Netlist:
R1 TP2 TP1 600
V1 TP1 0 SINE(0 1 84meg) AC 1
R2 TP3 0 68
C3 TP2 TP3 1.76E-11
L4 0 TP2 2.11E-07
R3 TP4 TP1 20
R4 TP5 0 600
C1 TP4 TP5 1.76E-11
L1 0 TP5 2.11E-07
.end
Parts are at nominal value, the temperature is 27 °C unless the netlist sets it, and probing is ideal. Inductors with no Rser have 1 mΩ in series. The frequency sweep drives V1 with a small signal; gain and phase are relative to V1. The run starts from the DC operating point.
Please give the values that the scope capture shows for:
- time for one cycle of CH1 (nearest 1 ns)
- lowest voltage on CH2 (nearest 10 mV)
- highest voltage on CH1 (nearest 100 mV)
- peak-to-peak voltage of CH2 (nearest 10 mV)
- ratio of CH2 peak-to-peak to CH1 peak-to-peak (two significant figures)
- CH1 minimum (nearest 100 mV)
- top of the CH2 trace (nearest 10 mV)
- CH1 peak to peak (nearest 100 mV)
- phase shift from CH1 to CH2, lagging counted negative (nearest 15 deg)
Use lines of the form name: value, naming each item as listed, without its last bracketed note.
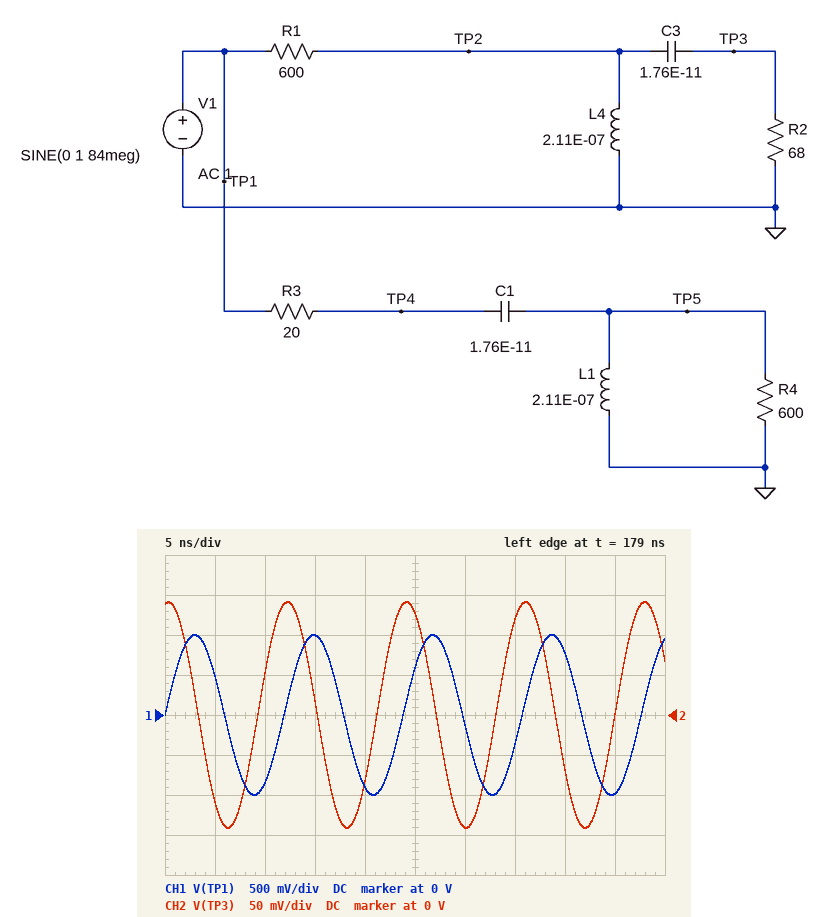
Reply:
time for one cycle of CH1: 12 ns
lowest voltage on CH2: -140 mV
highest voltage on CH1: 1.0 V
peak-to-peak voltage of CH2: 280 mV
ratio of CH2 peak-to-peak to CH1 peak-to-peak: 0.14
CH1 minimum: -1.0 V
top of the CH2 trace: 140 mV
CH1 peak to peak: 2.0 V
phase shift from CH1 to CH2, lagging counted negative: 75 deg
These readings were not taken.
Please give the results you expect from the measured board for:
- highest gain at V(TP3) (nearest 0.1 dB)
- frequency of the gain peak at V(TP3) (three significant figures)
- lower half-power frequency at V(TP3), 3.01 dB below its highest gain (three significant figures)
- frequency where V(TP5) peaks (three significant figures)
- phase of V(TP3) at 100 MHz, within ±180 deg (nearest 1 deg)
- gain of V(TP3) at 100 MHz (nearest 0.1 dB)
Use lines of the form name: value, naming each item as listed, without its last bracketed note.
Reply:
highest gain at V(TP3): -16.8 dB
frequency of the gain peak at V(TP3): 92.9 MHz
lower half-power frequency at V(TP3), 3.01 dB below its highest gain: 65.8 MHz
frequency where V(TP5) peaks: 84.0 MHz
phase of V(TP3) at 100 MHz, within ±180 deg: 57 deg
gain of V(TP3) at 100 MHz: -16.9 dB
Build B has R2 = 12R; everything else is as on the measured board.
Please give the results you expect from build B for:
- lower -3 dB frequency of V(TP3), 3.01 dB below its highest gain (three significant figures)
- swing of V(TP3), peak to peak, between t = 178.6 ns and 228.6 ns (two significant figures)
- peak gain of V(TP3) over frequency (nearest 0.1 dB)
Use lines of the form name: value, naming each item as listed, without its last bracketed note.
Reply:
lower -3 dB frequency of V(TP3), 3.01 dB below its highest gain: 73.3 MHz
swing of V(TP3), peak to peak, between t = 178.6 ns and 228.6 ns: 140 mV
peak gain of V(TP3) over frequency: -23.3 dB
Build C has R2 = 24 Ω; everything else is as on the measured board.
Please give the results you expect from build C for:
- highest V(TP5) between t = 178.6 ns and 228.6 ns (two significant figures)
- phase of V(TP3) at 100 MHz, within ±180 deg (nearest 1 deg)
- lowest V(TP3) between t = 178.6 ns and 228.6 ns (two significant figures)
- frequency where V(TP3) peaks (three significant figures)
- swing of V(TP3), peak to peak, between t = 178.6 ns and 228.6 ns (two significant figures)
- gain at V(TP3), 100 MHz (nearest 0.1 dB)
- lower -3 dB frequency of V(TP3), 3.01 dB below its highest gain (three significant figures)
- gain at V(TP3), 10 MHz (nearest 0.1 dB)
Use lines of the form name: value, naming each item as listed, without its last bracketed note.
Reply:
highest V(TP5) between t = 178.6 ns and 228.6 ns: 2.7 V
phase of V(TP3) at 100 MHz, within ±180 deg: 43 deg
lowest V(TP3) between t = 178.6 ns and 228.6 ns: -100 mV
frequency where V(TP3) peaks: 84.3 MHz
swing of V(TP3), peak to peak, between t = 178.6 ns and 228.6 ns: 200 mV
gain at V(TP3), 100 MHz: -21.7 dB
lower -3 dB frequency of V(TP3), 3.01 dB below its highest gain: 70.8 MHz
gain at V(TP3), 10 MHz: -64.5 dB
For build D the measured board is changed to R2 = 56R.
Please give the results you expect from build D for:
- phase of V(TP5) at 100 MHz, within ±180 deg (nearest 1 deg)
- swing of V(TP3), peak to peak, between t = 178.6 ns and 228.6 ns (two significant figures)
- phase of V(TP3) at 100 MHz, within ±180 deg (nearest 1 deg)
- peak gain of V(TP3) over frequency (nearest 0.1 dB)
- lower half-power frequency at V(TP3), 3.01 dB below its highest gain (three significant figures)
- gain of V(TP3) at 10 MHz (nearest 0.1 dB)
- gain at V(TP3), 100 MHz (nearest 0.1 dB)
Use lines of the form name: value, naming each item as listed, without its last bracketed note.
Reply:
phase of V(TP5) at 100 MHz, within ±180 deg: 41 deg
swing of V(TP3), peak to peak, between t = 178.6 ns and 228.6 ns: 270 mV
phase of V(TP3) at 100 MHz, within ±180 deg: 54 deg
peak gain of V(TP3) over frequency: -17.3 dB
lower half-power frequency at V(TP3), 3.01 dB below its highest gain: 66.6 MHz
gain of V(TP3) at 10 MHz: -57.2 dB
gain at V(TP3), 100 MHz: -17.6 dB
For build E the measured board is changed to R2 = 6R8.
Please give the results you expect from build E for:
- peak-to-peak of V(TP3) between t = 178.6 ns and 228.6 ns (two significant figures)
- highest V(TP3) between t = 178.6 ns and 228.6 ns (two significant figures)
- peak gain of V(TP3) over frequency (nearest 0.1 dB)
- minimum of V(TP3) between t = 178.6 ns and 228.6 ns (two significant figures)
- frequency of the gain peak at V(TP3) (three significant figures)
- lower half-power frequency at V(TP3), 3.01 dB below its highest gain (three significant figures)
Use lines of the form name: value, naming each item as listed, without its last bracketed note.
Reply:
peak-to-peak of V(TP3) between t = 178.6 ns and 228.6 ns: 93 mV
highest V(TP3) between t = 178.6 ns and 228.6 ns: 46 mV
peak gain of V(TP3) over frequency: -26.7 dB
minimum of V(TP3) between t = 178.6 ns and 228.6 ns: -46 mV
frequency of the gain peak at V(TP3): 83.4 MHz
lower half-power frequency at V(TP3), 3.01 dB below its highest gain: 74.6 MHz
